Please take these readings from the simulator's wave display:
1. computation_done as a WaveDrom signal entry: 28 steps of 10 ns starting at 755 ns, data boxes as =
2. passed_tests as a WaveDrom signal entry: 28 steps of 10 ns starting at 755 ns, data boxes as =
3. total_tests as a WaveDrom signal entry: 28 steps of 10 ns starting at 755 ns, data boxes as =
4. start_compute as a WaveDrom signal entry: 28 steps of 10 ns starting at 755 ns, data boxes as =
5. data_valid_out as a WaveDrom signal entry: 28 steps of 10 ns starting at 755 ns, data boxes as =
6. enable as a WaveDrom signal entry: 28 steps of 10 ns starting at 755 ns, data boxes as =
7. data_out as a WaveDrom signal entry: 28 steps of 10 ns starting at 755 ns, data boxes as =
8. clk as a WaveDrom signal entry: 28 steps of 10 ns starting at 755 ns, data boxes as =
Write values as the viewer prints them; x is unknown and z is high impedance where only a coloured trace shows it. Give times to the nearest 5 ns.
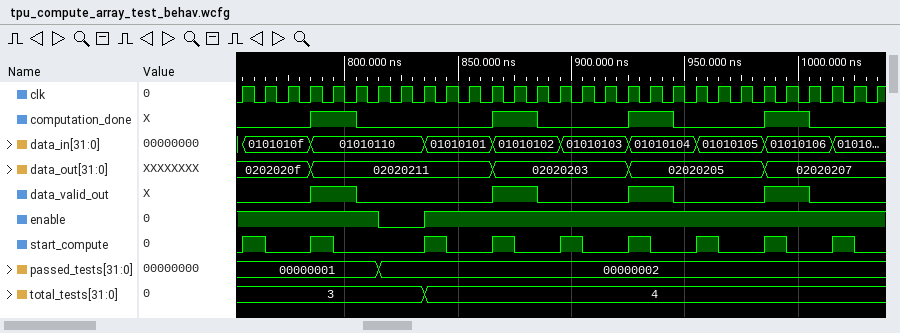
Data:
{name: 'computation_done', wave: '0..1.0.....1.0...1.0...1.0..'}
{name: 'passed_tests', wave: '=.....=.....................', data: '00000001 00000002'}
{name: 'total_tests', wave: '=.......=...................', data: '3 4'}
{name: 'start_compute', wave: '10.10...10.10.10.10.10.10.10'}
{name: 'data_valid_out', wave: '0..1.0.....1.0...1.0...1.0..'}
{name: 'enable', wave: '1.....0.1...................'}
{name: 'data_out', wave: '=..=.......=.....=.....=....', data: '0202020f 02020211 02020203 02020205 02020207'}
{name: 'clk', wave: 'p...........................'}
